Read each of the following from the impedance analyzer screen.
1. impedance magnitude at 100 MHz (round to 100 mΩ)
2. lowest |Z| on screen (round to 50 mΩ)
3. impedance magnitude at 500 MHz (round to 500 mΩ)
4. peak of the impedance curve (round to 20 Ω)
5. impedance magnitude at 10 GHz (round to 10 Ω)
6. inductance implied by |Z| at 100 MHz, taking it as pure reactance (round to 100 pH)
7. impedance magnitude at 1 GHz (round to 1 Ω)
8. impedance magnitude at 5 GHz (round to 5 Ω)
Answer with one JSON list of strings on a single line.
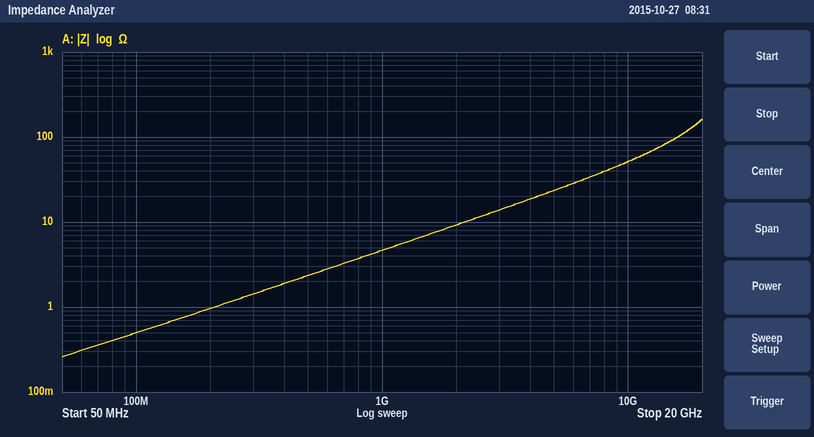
["500 mΩ", "250 mΩ", "2.5 Ω", "160 Ω", "50 Ω", "800 pH", "5 Ω", "25 Ω"]
